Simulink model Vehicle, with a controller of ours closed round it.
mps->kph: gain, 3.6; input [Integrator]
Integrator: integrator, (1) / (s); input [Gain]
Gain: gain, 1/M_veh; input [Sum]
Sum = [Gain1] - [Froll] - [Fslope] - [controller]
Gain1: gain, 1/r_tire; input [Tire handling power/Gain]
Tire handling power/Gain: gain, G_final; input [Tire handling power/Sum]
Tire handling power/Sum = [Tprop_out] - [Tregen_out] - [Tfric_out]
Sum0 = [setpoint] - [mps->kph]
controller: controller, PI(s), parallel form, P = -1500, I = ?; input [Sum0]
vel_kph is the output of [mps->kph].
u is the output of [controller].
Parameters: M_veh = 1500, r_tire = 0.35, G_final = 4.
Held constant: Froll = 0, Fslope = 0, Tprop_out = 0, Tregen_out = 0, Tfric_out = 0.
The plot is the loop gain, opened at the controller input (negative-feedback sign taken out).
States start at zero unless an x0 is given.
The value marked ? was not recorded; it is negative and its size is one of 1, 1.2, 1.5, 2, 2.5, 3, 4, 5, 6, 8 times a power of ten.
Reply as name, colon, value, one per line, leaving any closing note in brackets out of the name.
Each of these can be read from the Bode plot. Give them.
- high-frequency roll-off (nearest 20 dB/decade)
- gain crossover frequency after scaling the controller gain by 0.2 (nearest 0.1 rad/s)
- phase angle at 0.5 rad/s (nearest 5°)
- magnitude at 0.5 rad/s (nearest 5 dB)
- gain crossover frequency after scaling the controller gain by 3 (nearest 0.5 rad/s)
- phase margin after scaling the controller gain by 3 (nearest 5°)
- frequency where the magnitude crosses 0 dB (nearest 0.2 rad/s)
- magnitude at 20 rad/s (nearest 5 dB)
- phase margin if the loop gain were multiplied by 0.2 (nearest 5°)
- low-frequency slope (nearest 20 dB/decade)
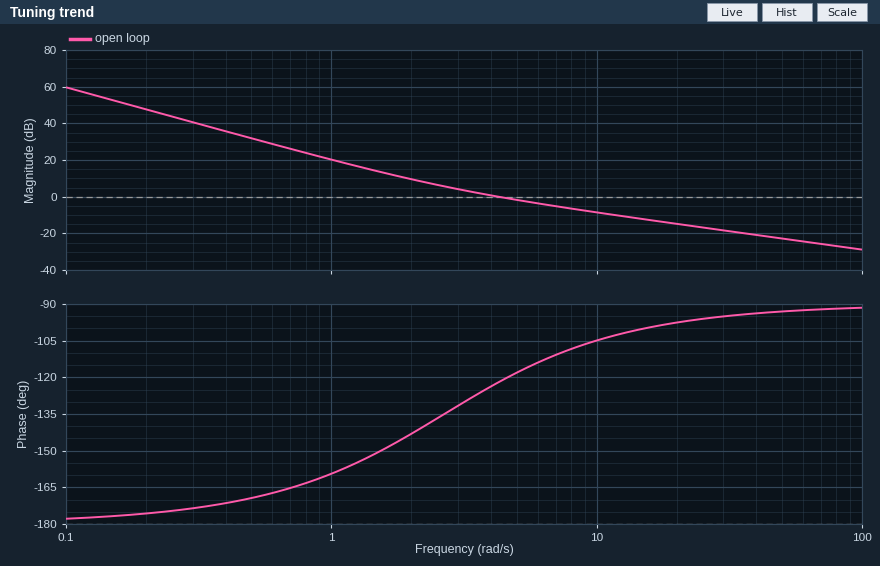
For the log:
high-frequency roll-off: -20 dB/decade
gain crossover frequency after scaling the controller gain by 0.2: 1.5 rad/s
phase angle at 0.5 rad/s: -170°
magnitude at 0.5 rad/s: 30 dB
gain crossover frequency after scaling the controller gain by 3: 11.0 rad/s
phase margin after scaling the controller gain by 3: 75°
frequency where the magnitude crosses 0 dB: 4.2 rad/s
magnitude at 20 rad/s: -15 dB
phase margin if the loop gain were multiplied by 0.2: 30°
low-frequency slope: -40 dB/decade
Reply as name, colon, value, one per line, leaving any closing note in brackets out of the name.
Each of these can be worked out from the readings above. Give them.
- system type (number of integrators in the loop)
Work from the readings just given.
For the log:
system type: 2
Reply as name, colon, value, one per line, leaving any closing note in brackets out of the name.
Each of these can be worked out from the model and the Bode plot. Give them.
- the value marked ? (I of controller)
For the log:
the value marked ?: -4000
